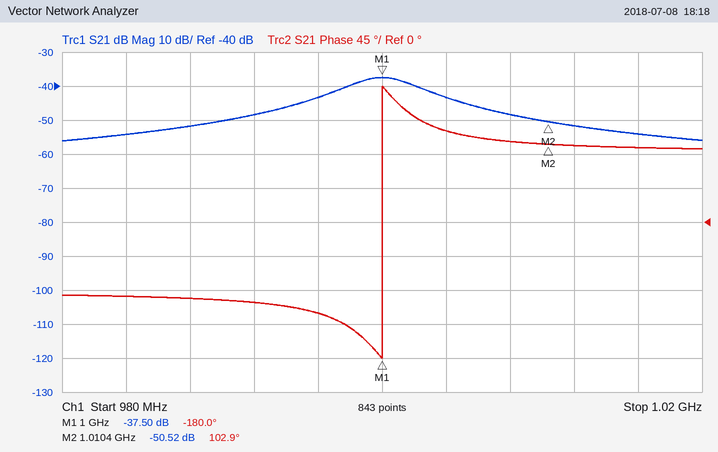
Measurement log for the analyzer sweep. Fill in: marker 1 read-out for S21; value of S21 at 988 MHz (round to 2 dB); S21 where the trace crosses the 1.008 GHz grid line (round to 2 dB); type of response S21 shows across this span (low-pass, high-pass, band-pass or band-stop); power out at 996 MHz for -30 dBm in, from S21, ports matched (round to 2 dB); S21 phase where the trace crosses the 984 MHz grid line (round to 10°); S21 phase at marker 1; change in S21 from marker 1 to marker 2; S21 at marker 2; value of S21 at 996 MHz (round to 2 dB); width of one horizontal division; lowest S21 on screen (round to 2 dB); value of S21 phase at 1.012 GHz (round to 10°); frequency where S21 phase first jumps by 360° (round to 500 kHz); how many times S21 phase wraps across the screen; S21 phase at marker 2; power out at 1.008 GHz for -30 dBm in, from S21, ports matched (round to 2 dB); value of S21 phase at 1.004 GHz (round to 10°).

-37.50 dB
-52 dB
-48 dB
band-pass
-74 dBm
-100°
-180.0°
-13.02 dB
-50.52 dB
-44 dB
4 MHz
-56 dB
100°
1.0000 GHz
1
102.9°
-78 dBm
120°
